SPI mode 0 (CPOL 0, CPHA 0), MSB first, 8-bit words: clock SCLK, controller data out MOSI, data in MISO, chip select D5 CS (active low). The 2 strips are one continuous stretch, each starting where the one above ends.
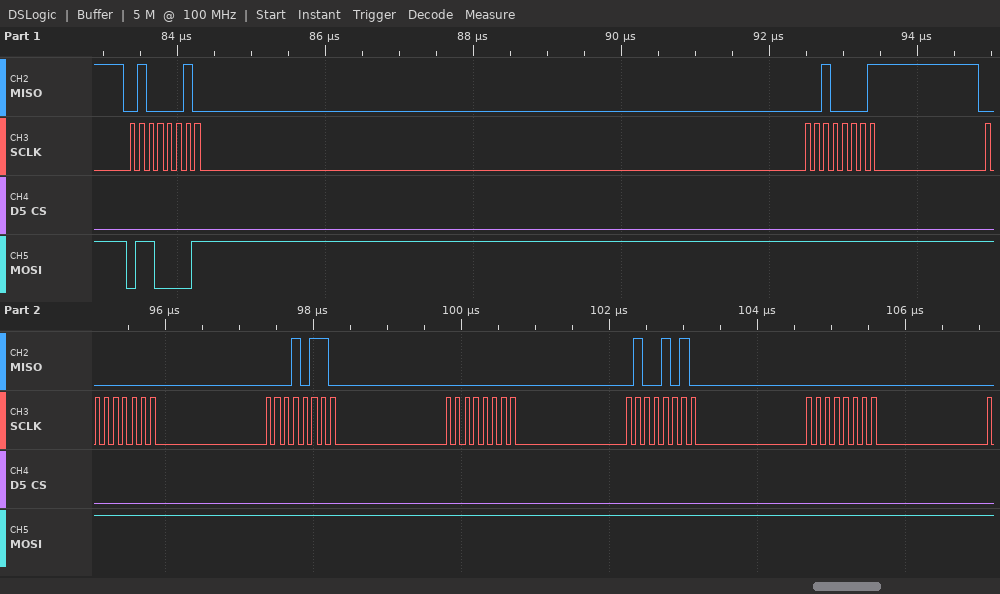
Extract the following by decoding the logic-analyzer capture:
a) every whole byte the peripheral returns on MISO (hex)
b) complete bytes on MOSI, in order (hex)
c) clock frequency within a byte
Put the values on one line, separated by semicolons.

42 21 00 16 00 4A 00; 61 FF FF FF FF FF FF; 8 MHz
